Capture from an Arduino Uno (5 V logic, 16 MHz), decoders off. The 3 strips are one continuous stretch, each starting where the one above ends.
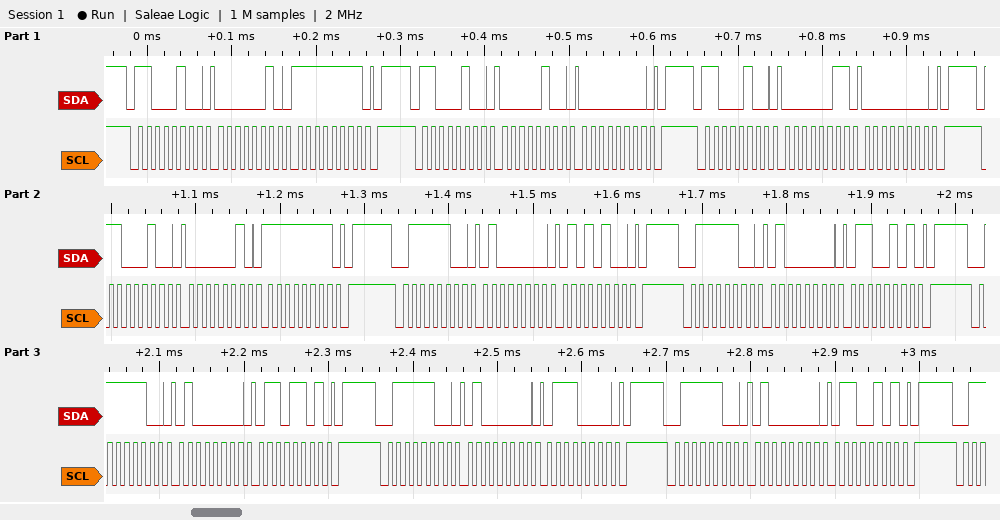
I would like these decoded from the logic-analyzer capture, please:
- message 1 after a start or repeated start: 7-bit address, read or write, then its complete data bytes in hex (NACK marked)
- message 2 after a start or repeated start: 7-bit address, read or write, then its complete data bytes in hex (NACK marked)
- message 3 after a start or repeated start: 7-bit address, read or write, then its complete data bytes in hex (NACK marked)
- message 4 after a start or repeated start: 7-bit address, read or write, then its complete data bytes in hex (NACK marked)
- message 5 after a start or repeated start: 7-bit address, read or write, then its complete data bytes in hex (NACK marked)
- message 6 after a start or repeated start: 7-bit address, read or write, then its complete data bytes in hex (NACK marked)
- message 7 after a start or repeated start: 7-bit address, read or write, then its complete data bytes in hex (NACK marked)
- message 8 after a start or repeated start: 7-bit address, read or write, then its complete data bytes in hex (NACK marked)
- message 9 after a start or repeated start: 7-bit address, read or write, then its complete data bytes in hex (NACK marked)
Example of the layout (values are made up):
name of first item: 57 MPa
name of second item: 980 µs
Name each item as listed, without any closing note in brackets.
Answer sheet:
message 1 after a start or repeated start: 7-bit address, read or write, then its complete data bytes in hex: 0x62 write: 02 FF
message 2 after a start or repeated start: 7-bit address, read or write, then its complete data bytes in hex: 0x62 write: 04 00
message 3 after a start or repeated start: 7-bit address, read or write, then its complete data bytes in hex: 0x62 write: 03 00
message 4 after a start or repeated start: 7-bit address, read or write, then its complete data bytes in hex: 0x62 write: 02 FF
message 5 after a start or repeated start: 7-bit address, read or write, then its complete data bytes in hex: 0x3E write: 40 54
message 6 after a start or repeated start: 7-bit address, read or write, then its complete data bytes in hex: 0x3E write: 40 65
message 7 after a start or repeated start: 7-bit address, read or write, then its complete data bytes in hex: 0x3E write: 40 6D
message 8 after a start or repeated start: 7-bit address, read or write, then its complete data bytes in hex: 0x3E write: 40 70
message 9 after a start or repeated start: 7-bit address, read or write, then its complete data bytes in hex: 0x3E write: 40 65
